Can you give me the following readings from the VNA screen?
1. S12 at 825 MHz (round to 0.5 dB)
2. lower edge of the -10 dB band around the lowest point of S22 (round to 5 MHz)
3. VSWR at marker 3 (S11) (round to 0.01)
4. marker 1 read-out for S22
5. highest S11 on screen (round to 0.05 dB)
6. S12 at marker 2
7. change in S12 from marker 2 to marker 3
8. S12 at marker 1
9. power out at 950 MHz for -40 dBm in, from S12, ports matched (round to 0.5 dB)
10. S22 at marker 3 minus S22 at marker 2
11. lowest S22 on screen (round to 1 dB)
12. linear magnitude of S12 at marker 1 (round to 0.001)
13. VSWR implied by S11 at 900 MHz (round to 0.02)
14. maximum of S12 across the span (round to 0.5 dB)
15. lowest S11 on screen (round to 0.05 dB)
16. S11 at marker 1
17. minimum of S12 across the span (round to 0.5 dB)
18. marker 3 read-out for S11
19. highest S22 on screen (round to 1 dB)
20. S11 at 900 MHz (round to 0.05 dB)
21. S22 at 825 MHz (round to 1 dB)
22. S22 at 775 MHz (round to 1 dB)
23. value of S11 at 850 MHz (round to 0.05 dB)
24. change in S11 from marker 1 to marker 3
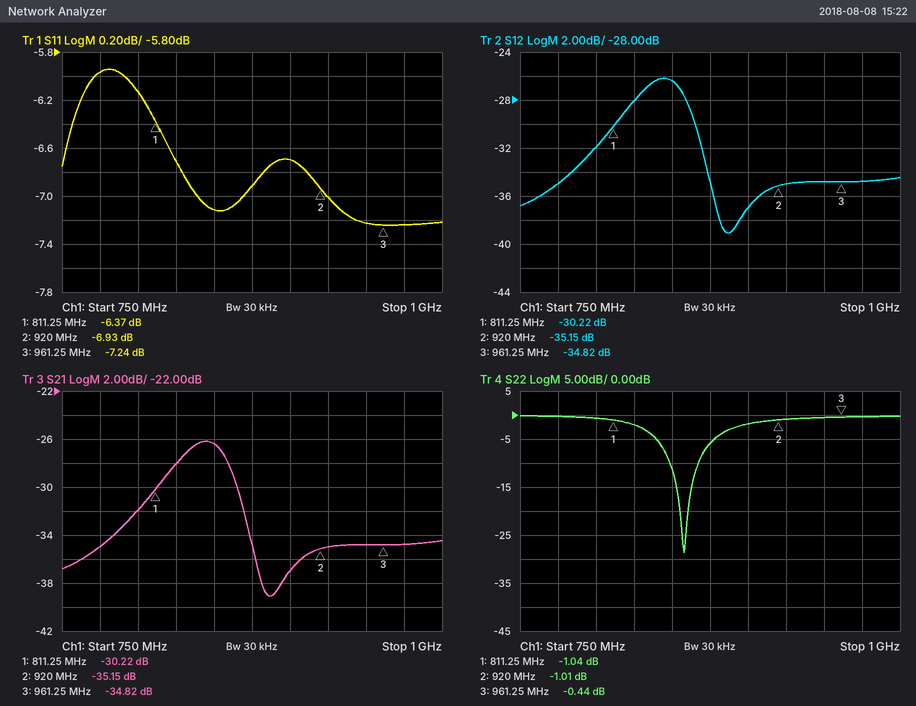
-28.0 dB
850 MHz
2.54
-1.04 dB
-5.95 dB
-35.15 dB
0.33 dB
-30.22 dB
-75.0 dBm
0.57 dB
-29 dB
0.031
2.72
-26.0 dB
-7.25 dB
-6.37 dB
-39.0 dB
-7.24 dB
0 dB
-6.70 dB
-2 dB
0 dB
-7.10 dB
-0.87 dB
